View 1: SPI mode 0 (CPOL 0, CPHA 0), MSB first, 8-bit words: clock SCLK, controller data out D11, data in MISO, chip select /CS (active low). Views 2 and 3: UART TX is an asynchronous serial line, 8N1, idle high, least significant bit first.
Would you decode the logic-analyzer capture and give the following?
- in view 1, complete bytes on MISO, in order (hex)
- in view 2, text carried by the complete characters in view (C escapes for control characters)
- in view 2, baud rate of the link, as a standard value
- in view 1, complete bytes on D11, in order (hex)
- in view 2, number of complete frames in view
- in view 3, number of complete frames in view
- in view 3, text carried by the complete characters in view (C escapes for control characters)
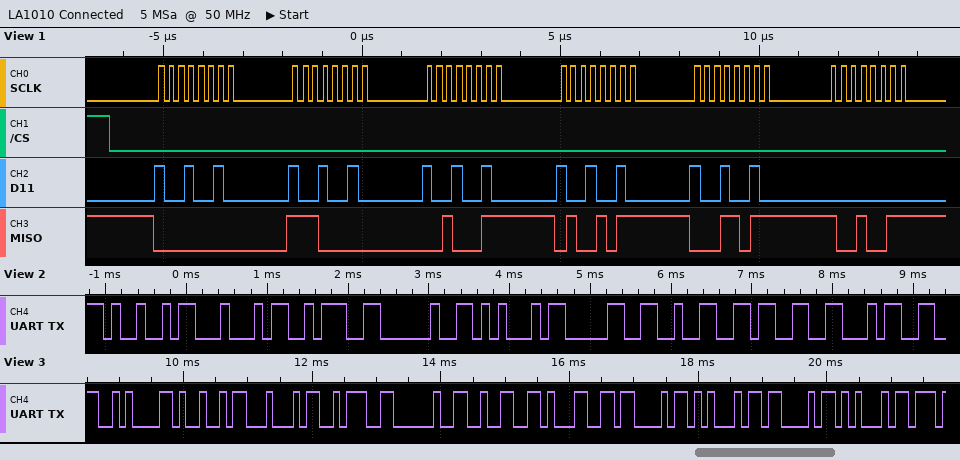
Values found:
00 E0 23 4B 1B 93
"ID: E0234"
9600 baud
92 92 92 92 92 00
9
11
"\nID: 21CECE"
